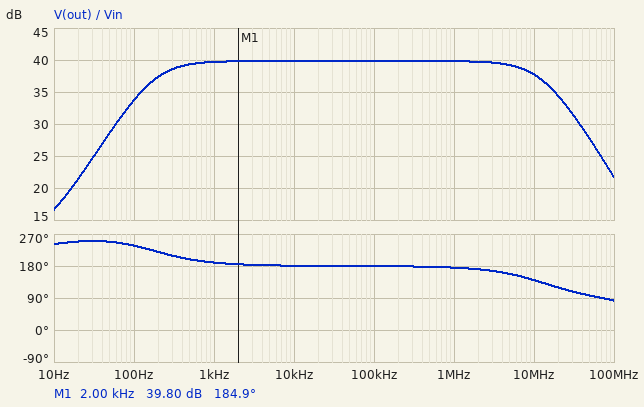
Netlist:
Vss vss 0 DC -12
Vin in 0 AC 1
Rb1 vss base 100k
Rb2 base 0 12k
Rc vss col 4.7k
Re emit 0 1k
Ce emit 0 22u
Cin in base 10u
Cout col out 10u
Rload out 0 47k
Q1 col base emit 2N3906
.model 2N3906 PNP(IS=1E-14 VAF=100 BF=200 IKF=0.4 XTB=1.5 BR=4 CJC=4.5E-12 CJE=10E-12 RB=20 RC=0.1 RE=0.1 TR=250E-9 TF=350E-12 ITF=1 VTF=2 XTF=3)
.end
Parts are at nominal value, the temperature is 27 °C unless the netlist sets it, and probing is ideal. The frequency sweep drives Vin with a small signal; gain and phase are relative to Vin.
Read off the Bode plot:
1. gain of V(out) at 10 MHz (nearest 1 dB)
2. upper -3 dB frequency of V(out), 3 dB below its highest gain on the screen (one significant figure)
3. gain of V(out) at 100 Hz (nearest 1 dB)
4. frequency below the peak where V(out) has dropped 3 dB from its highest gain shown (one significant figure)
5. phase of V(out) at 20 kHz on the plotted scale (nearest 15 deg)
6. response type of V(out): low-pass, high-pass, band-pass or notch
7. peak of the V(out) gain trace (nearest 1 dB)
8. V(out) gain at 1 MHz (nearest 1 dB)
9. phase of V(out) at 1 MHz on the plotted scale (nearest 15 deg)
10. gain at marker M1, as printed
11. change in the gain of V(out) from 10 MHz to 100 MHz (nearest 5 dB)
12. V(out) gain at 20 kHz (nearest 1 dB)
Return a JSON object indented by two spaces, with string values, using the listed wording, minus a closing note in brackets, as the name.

{
  "gain of V(out) at 10 MHz": "38 dB",
  "upper -3 dB frequency of V(out), 3 dB below its highest gain on the screen": "10 MHz",
  "gain of V(out) at 100 Hz": "34 dB",
  "frequency below the peak where V(out) has dropped 3 dB from its highest gain shown": "200 Hz",
  "phase of V(out) at 20 kHz on the plotted scale": "180 deg",
  "response type of V(out): low-pass, high-pass, band-pass or notch": "band-pass",
  "peak of the V(out) gain trace": "40 dB",
  "V(out) gain at 1 MHz": "40 dB",
  "phase of V(out) at 1 MHz on the plotted scale": "180 deg",
  "gain at marker M1, as printed": "39.80 dB",
  "change in the gain of V(out) from 10 MHz to 100 MHz": "-15 dB",
  "V(out) gain at 20 kHz": "40 dB"
}
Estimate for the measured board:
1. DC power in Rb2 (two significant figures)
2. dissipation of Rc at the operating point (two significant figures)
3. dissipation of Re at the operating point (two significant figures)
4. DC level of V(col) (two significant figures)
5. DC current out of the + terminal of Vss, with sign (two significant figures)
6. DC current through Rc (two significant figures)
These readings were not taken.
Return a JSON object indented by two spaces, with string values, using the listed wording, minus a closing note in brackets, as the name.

{
  "DC power in Rb2": "130 µW",
  "dissipation of Rc at the operating point": "1.8 mW",
  "dissipation of Re at the operating point": "380 µW",
  "DC level of V(col)": "-9.1 V",
  "DC current out of the + terminal of Vss, with sign": "-720 µA",
  "DC current through Rc": "610 µA"
}
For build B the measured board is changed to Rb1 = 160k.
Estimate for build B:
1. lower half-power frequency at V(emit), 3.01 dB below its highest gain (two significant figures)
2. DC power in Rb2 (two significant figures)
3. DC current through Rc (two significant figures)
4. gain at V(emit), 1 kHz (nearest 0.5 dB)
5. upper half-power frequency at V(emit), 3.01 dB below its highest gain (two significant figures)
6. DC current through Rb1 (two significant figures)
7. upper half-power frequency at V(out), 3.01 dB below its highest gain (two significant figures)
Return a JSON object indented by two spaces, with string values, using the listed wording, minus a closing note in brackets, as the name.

{
  "lower half-power frequency at V(emit), 3.01 dB below its highest gain": "1.4 Hz",
  "DC power in Rb2": "57 µW",
  "DC current through Rc": "210 µA",
  "gain at V(emit), 1 kHz": "-24.5 dB",
  "upper half-power frequency at V(emit), 3.01 dB below its highest gain": "70 Hz",
  "DC current through Rb1": "70 µA",
  "upper half-power frequency at V(out), 3.01 dB below its highest gain": "17 MHz"
}
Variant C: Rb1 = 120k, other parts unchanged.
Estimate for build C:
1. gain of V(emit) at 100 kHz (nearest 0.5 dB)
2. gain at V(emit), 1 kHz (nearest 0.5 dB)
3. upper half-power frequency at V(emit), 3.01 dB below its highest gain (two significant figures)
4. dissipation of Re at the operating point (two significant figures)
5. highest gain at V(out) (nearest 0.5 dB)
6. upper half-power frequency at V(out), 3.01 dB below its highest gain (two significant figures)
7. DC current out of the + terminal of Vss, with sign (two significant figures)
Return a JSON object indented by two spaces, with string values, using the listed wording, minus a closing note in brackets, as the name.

{
  "gain of V(emit) at 100 kHz": "-58.5 dB",
  "gain at V(emit), 1 kHz": "-18.5 dB",
  "upper half-power frequency at V(emit), 3.01 dB below its highest gain": "130 Hz",
  "dissipation of Re at the operating point": "190 µW",
  "highest gain at V(out)": "37.0 dB",
  "upper half-power frequency at V(out), 3.01 dB below its highest gain": "14 MHz",
  "DC current out of the + terminal of Vss, with sign": "-530 µA"
}
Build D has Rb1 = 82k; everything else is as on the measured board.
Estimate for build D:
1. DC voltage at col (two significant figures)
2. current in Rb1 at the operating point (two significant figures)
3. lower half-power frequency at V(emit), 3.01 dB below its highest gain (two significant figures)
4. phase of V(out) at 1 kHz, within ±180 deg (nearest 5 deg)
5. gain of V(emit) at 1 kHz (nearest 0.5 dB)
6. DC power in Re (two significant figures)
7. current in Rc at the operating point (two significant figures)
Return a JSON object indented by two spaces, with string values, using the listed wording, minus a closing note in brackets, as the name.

{
  "DC voltage at col": "-8.1 V",
  "current in Rb1 at the operating point": "130 µA",
  "lower half-power frequency at V(emit), 3.01 dB below its highest gain": "1.6 Hz",
  "phase of V(out) at 1 kHz, within ±180 deg": "-165 deg",
  "gain of V(emit) at 1 kHz": "-13.0 dB",
  "DC power in Re": "710 µW",
  "current in Rc at the operating point": "840 µA"
}
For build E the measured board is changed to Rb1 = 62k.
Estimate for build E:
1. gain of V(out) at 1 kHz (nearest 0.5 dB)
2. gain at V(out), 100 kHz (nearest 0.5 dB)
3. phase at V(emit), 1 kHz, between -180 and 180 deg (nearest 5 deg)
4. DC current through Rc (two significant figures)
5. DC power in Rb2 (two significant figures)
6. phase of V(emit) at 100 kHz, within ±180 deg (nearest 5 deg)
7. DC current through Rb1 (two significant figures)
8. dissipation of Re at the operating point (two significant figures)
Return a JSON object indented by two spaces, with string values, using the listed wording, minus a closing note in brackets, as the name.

{
  "gain of V(out) at 1 kHz": "45.0 dB",
  "gain at V(out), 100 kHz": "45.5 dB",
  "phase at V(emit), 1 kHz, between -180 and 180 deg": "-70 deg",
  "DC current through Rc": "1.2 mA",
  "DC power in Rb2": "300 µW",
  "phase of V(emit) at 100 kHz, within ±180 deg": "-90 deg",
  "DC current through Rb1": "160 µA",
  "dissipation of Re at the operating point": "1.5 mW"
}
